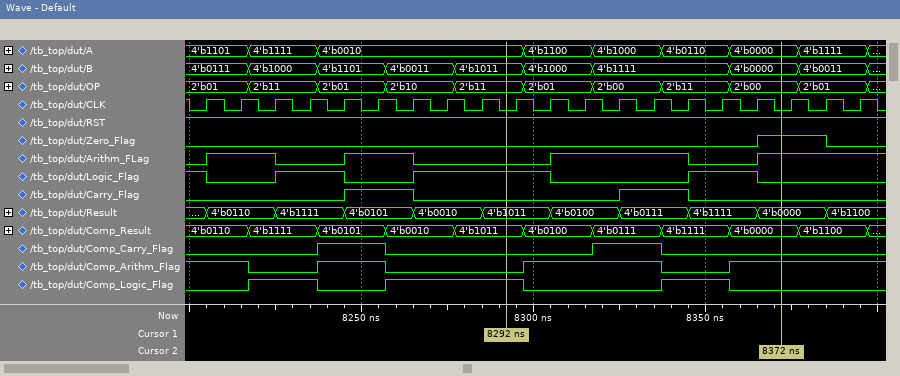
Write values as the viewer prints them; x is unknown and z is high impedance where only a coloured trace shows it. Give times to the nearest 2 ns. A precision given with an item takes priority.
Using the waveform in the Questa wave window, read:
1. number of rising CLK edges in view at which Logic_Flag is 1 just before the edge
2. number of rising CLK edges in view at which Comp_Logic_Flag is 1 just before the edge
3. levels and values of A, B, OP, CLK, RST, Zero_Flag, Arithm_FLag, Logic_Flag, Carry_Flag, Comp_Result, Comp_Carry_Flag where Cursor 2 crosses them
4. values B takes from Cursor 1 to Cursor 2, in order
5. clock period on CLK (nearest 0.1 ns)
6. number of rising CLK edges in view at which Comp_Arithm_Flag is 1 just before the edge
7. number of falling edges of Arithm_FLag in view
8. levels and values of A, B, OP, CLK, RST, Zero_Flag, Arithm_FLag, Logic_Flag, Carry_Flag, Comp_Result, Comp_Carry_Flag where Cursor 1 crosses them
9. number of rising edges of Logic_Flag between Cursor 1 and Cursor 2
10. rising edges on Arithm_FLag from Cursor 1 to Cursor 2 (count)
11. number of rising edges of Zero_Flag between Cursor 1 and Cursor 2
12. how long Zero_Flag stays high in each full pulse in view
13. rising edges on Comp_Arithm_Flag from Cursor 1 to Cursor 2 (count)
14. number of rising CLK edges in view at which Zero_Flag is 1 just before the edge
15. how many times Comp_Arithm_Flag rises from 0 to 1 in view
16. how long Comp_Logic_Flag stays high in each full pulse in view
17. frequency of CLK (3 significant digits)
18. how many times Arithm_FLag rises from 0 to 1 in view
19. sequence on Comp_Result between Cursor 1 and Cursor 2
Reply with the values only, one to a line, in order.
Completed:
9
8
A=4'b0000, B=4'b0000, OP=2'b00, CLK=0, RST=1, Zero_Flag=1, Arithm_FLag=1, Logic_Flag=0, Carry_Flag=0, Comp_Result=4'b0000, Comp_Carry_Flag=0
4'b1011, 4'b1000, 4'b1111, 4'b0000
10 ns
12
3
A=4'b0010, B=4'b1011, OP=2'b11, CLK=0, RST=1, Zero_Flag=0, Arithm_FLag=0, Logic_Flag=1, Carry_Flag=0, Comp_Result=4'b1011, Comp_Carry_Flag=0
1
2
1
20 ns
2
2
3
20 ns, 40 ns, 20 ns
100 MHz
4
4'b1011, 4'b0100, 4'b0111, 4'b1111, 4'b0000
